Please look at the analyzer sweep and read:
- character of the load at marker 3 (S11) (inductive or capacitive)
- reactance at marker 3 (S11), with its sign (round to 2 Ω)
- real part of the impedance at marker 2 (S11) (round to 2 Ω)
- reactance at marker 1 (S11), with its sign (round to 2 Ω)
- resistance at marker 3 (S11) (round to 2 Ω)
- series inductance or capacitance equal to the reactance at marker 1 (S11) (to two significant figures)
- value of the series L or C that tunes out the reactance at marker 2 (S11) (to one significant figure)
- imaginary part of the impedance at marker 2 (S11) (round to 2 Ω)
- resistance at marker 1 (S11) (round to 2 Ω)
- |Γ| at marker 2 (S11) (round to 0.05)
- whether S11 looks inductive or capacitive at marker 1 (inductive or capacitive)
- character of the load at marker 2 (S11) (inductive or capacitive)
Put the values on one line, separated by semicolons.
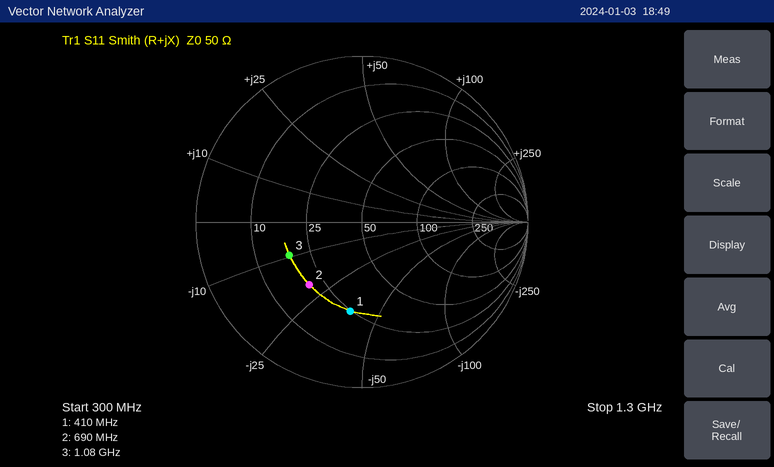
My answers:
capacitive; -10 Ω; 20 Ω; -38 Ω; 18 Ω; 10 pF; 5 nH; -20 Ω; 24 Ω; 0.50; capacitive; capacitive
